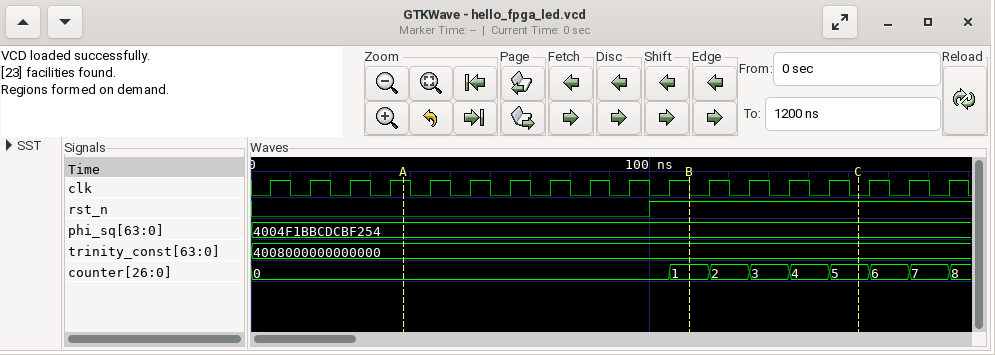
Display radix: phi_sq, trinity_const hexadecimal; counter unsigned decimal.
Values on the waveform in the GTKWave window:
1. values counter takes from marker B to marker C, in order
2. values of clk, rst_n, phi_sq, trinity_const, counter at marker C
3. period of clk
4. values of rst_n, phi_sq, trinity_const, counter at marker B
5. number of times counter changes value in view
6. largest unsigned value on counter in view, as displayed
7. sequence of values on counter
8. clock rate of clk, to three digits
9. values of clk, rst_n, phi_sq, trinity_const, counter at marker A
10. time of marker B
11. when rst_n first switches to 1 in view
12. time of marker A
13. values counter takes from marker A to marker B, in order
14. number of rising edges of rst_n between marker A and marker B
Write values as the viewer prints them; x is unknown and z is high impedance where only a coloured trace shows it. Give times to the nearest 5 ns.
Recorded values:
1, 2, 3, 4, 5
clk=0, rst_n=1, phi_sq=4004F1BBCDCBF254, trinity_const=4008000000000000, counter=5
10 ns
rst_n=1, phi_sq=4004F1BBCDCBF254, trinity_const=4008000000000000, counter=1
8
8
0, 1, 2, 3, 4, 5, 6, 7, 8
100 MHz
clk=1, rst_n=0, phi_sq=4004F1BBCDCBF254, trinity_const=4008000000000000, counter=0
110 ns
100 ns
40 ns
0, 1
1
